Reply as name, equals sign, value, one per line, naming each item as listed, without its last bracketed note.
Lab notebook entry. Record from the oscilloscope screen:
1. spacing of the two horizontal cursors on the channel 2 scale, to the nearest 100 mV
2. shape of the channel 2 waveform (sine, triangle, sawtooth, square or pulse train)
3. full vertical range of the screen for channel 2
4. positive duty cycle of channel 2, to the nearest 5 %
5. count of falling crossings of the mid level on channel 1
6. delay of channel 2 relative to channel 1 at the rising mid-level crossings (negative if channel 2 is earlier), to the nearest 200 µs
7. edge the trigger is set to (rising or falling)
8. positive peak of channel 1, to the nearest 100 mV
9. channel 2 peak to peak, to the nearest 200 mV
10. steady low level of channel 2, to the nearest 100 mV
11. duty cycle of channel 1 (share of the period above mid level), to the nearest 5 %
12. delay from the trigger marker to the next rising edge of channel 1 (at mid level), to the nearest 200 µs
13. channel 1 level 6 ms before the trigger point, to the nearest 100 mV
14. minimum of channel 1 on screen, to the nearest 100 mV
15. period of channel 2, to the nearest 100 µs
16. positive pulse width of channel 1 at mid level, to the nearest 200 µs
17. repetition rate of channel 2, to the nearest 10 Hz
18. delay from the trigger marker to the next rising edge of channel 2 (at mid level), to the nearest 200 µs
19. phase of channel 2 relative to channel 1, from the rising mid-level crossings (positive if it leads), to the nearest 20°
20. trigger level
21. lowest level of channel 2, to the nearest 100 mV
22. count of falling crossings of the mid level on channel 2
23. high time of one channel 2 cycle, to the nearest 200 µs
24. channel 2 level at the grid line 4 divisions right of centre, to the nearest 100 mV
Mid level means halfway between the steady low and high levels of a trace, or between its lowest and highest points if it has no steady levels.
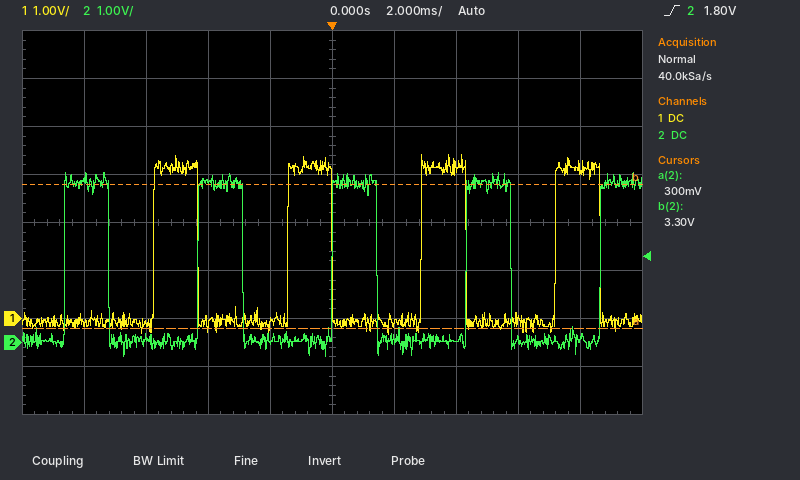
spacing of the two horizontal cursors on the channel 2 scale, to the nearest 100 mV = 3.0 V
shape of the channel 2 waveform = pulse train
full vertical range of the screen for channel 2 = 8 V
positive duty cycle of channel 2, to the nearest 5 % = 35 %
count of falling crossings of the mid level on channel 1 = 4
delay of channel 2 relative to channel 1 at the rising mid-level crossings (negative if channel 2 is earlier), to the nearest 200 µs = +1.4 ms
edge the trigger is set to = rising
positive peak of channel 1, to the nearest 100 mV = 3.4 V
channel 2 peak to peak, to the nearest 200 mV = 3.8 V
steady low level of channel 2, to the nearest 100 mV = 0.0 V
duty cycle of channel 1 (share of the period above mid level), to the nearest 5 % = 35 %
delay from the trigger marker to the next rising edge of channel 1 (at mid level), to the nearest 200 µs = 2.8 ms
channel 1 level 6 ms before the trigger point, to the nearest 100 mV = -100 mV
minimum of channel 1 on screen, to the nearest 100 mV = -300 mV
period of channel 2, to the nearest 100 µs = 4.3 ms
positive pulse width of channel 1 at mid level, to the nearest 200 µs = 1.4 ms
repetition rate of channel 2, to the nearest 10 Hz = 230 Hz
delay from the trigger marker to the next rising edge of channel 2 (at mid level), to the nearest 200 µs = 4.4 ms
phase of channel 2 relative to channel 1, from the rising mid-level crossings (positive if it leads), to the nearest 20° = -120°
trigger level = 1.80 V
lowest level of channel 2, to the nearest 100 mV = -300 mV
count of falling crossings of the mid level on channel 2 = 4
high time of one channel 2 cycle, to the nearest 200 µs = 1.4 ms
channel 2 level at the grid line 4 divisions right of centre, to the nearest 100 mV = 100 mV
